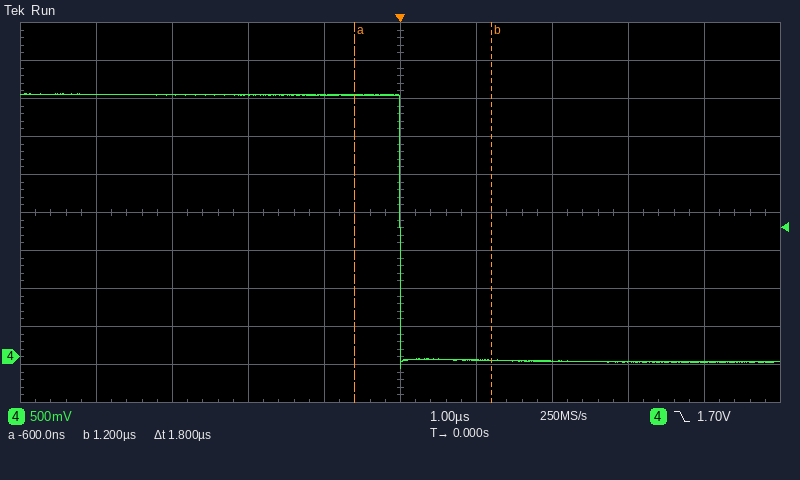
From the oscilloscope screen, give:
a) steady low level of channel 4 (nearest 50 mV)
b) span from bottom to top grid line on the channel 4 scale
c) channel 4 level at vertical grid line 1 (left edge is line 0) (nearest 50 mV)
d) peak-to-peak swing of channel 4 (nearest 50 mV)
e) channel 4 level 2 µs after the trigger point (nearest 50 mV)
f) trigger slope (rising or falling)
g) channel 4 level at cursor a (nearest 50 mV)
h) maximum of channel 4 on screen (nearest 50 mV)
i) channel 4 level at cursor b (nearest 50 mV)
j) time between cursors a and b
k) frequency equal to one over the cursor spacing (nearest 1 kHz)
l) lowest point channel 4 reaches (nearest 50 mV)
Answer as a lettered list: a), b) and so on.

a) -50 mV
b) 5 V
c) 3.45 V
d) 3.60 V
e) -50 mV
f) falling
g) 3.45 V
h) 3.45 V
i) -50 mV
j) 1.8 µs
k) 556 kHz
l) -150 mV
